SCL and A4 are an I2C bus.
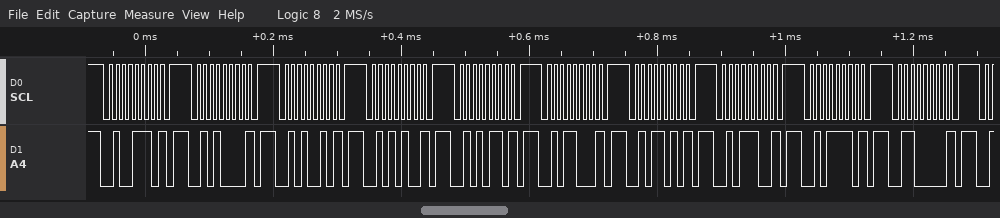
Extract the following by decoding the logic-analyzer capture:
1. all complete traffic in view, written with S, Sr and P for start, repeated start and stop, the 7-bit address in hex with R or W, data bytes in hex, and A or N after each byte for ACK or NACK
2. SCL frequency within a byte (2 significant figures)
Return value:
S 27W N P S 28W N P S 29W N P S 2AW N P S 2BW N P S 2CW N P S 2DW N P S 2EW N P S 2FW N P S 30W N P
100 kHz
